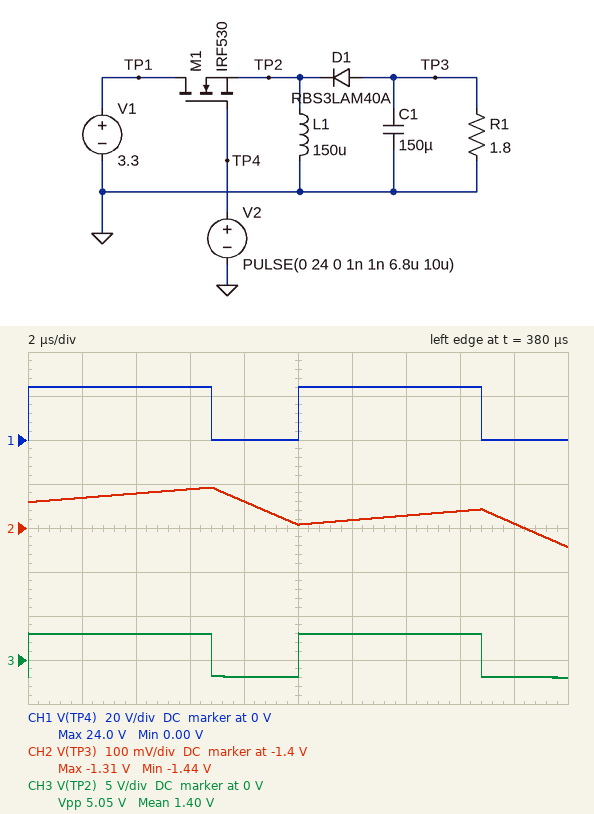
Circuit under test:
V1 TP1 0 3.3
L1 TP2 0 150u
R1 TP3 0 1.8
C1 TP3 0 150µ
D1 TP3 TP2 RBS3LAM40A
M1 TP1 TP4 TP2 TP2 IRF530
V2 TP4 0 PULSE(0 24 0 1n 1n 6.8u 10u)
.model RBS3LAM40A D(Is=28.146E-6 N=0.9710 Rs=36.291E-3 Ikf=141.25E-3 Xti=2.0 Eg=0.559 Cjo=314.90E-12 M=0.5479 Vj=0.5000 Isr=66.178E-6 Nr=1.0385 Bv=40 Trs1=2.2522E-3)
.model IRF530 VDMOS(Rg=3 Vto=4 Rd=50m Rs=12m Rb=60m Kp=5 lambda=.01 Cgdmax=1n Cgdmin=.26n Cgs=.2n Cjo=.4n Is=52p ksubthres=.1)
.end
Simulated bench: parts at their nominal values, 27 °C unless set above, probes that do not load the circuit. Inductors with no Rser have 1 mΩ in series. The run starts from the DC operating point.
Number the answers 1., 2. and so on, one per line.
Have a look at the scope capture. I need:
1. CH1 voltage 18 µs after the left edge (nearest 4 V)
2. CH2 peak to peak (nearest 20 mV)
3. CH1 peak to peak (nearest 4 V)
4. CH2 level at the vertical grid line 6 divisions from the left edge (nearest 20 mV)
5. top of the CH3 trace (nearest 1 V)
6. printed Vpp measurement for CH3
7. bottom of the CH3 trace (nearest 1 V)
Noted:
1. 0 V
2. 140 mV
3. 24 V
4. -1.38 V
5. 3 V
6. 5.05 V
7. -2 V
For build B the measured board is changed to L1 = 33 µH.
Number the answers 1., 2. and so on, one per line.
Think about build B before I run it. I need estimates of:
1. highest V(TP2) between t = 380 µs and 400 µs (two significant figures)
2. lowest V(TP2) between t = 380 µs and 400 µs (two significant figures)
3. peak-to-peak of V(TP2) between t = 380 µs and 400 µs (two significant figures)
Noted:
1. 2.5 V
2. -5.0 V
3. 7.4 V
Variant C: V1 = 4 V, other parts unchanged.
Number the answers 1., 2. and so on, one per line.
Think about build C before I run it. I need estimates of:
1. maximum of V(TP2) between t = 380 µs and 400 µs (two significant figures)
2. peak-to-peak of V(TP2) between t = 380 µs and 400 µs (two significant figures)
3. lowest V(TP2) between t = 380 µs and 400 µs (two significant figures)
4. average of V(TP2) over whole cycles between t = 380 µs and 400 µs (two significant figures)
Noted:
1. 3.7 V
2. 6.0 V
3. -2.4 V
4. 1.7 V
